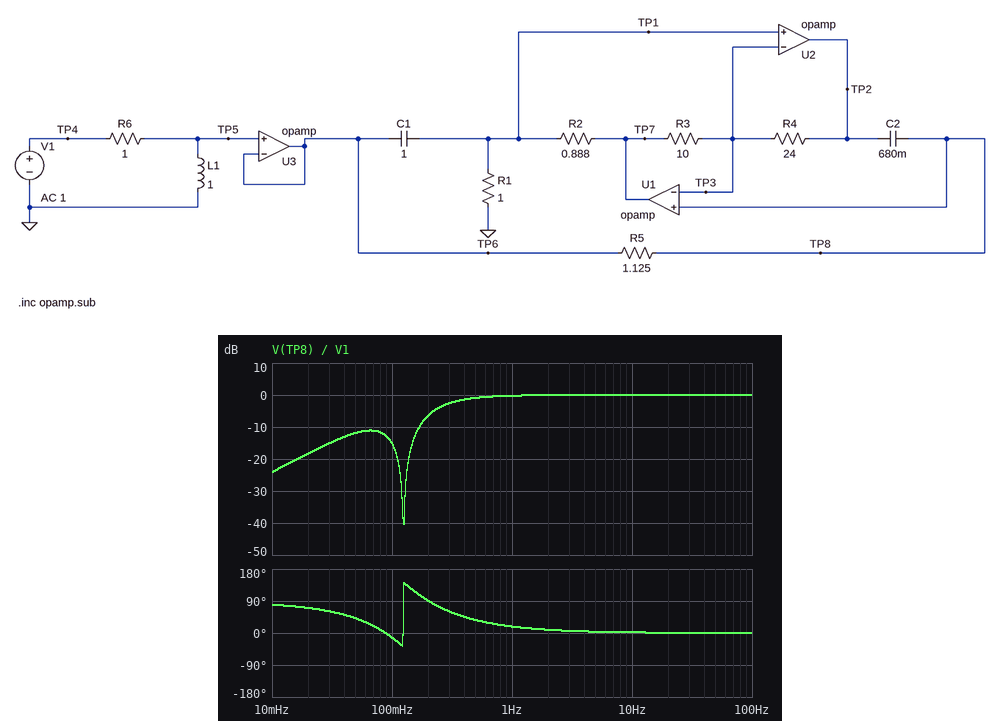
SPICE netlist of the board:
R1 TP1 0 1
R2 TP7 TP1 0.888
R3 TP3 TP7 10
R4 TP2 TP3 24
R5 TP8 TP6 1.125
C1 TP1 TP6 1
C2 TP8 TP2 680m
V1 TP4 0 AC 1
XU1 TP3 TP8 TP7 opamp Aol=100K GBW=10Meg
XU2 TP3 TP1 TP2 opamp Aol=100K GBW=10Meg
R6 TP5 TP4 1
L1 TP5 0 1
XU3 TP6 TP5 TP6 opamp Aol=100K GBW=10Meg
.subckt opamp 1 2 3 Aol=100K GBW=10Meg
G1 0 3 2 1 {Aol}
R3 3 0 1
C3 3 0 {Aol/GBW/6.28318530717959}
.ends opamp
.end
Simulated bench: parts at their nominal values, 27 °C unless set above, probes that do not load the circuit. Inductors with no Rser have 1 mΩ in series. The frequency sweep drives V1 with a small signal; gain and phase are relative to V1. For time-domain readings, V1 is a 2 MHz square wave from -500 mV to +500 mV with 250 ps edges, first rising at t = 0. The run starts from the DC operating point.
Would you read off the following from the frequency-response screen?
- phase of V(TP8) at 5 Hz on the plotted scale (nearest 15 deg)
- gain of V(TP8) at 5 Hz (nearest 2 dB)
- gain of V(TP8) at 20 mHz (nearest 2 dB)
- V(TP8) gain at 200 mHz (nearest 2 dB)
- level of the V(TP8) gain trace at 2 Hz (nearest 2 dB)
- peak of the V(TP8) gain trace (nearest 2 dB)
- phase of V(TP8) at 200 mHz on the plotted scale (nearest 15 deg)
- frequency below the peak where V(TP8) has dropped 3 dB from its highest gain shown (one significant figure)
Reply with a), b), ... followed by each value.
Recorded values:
a) 0 deg
b) 0 dB
c) -18 dB
d) -6 dB
e) 0 dB
f) 0 dB
g) 90 deg
h) 300 mHz
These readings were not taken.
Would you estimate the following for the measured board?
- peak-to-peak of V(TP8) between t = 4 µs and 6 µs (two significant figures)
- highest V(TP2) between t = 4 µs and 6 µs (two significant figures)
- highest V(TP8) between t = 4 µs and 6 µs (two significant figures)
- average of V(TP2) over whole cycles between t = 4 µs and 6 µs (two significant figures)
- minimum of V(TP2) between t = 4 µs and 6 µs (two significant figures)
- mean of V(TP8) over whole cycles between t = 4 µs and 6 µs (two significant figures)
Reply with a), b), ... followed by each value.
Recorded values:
a) 1.3 V
b) 1.2 V
c) 1.2 V
d) 500 mV
e) -160 mV
f) 500 mV
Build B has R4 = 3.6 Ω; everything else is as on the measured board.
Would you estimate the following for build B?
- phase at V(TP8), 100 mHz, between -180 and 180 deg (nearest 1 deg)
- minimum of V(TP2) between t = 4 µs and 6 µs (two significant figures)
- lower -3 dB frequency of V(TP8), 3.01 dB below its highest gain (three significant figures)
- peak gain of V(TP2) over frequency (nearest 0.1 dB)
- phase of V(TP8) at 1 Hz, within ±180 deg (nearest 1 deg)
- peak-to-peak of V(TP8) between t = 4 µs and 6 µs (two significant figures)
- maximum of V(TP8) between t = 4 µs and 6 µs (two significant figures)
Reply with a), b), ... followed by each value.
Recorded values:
a) 48 deg
b) -110 mV
c) 426 mHz
d) 0.2 dB
e) 19 deg
f) 1.2 V
g) 1.1 V
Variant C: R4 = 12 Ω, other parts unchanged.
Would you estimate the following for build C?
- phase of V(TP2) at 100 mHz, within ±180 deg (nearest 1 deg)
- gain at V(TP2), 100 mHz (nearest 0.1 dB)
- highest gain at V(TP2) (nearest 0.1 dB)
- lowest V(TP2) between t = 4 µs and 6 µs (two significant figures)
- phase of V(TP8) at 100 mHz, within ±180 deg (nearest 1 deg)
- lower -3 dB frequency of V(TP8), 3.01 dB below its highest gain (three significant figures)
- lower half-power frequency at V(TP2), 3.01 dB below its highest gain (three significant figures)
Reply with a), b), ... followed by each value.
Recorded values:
a) -159 deg
b) -12.3 dB
c) 0.6 dB
d) -150 mV
e) 21 deg
f) 309 mHz
g) 161 mHz
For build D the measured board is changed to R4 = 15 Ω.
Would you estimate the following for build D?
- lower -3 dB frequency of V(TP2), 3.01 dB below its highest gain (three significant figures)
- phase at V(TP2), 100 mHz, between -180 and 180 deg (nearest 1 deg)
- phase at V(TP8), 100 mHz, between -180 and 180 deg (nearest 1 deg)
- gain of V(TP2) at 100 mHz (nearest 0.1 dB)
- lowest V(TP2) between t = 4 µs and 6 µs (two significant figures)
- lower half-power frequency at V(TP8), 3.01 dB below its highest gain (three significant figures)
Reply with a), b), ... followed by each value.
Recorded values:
a) 136 mHz
b) -169 deg
c) 11 deg
d) -7.0 dB
e) -150 mV
f) 297 mHz
